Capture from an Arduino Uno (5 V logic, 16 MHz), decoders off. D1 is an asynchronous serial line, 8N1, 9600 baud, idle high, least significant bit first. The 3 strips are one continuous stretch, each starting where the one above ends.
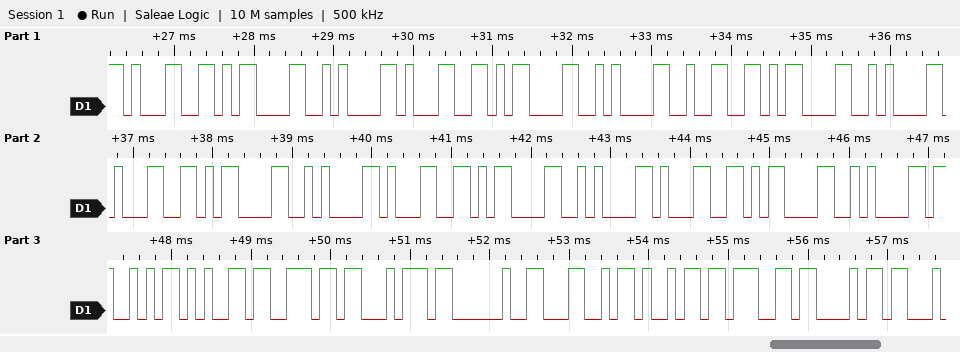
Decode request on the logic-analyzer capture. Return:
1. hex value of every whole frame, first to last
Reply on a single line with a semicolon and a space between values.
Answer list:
31 0D 0A 31 0D 0A 32 0D 0A 31 0D 0A 31 0D 0A 31 0D 0A 53 65 6E 74 20 4C 69 67 68
